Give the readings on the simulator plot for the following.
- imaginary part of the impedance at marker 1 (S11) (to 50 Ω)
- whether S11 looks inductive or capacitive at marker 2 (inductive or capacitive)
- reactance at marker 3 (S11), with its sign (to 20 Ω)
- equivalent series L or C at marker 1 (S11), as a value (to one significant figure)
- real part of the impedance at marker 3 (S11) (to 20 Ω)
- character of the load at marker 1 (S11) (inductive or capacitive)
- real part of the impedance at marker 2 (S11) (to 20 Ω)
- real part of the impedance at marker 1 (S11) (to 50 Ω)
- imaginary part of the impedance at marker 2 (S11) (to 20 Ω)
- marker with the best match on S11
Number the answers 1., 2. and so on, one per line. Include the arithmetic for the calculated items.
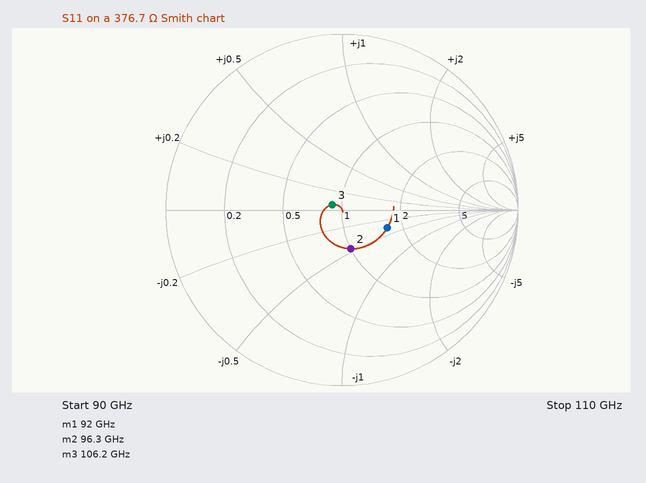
1. -150 Ω
2. capacitive
3. +20 Ω
4. C = 1/(2π × 92 GHz × 150 Ω) ≈ 11.5 fF, so 10 fF to one significant figure
5. 340 Ω
6. capacitive
7. 380 Ω
8. 600 Ω
9. -180 Ω
10. marker 3
